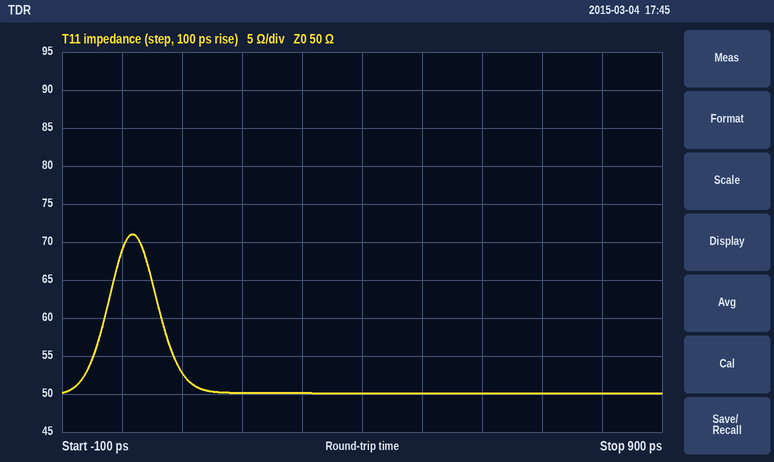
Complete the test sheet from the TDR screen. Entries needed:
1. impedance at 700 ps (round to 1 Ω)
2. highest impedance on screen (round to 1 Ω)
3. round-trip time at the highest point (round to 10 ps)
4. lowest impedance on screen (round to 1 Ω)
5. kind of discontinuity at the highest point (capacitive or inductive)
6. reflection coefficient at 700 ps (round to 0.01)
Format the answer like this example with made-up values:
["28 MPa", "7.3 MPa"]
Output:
["50 Ω", "71 Ω", "20 ps", "50 Ω", "inductive", "0.00"]
